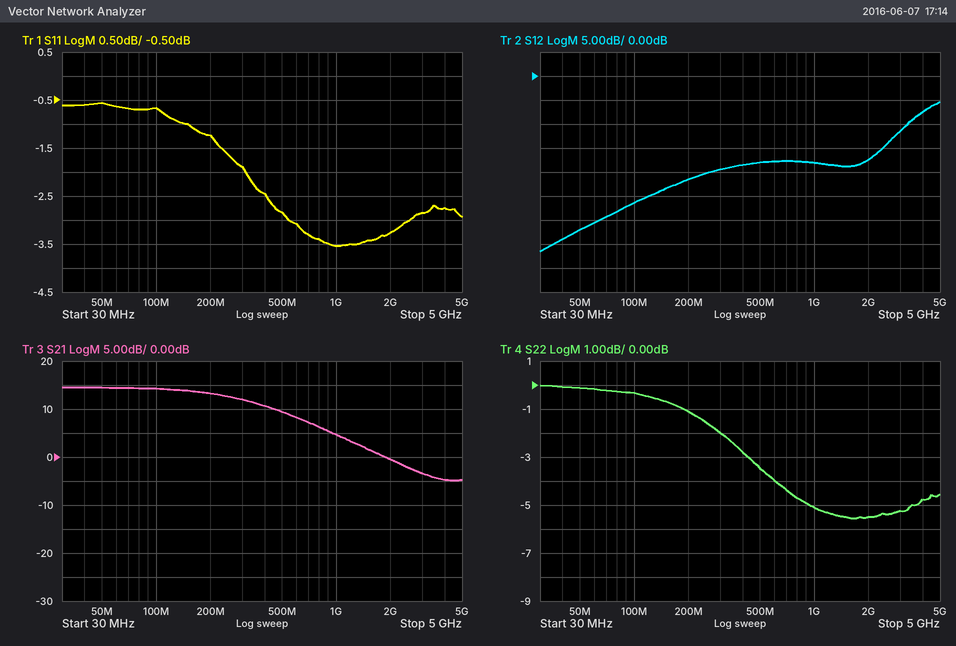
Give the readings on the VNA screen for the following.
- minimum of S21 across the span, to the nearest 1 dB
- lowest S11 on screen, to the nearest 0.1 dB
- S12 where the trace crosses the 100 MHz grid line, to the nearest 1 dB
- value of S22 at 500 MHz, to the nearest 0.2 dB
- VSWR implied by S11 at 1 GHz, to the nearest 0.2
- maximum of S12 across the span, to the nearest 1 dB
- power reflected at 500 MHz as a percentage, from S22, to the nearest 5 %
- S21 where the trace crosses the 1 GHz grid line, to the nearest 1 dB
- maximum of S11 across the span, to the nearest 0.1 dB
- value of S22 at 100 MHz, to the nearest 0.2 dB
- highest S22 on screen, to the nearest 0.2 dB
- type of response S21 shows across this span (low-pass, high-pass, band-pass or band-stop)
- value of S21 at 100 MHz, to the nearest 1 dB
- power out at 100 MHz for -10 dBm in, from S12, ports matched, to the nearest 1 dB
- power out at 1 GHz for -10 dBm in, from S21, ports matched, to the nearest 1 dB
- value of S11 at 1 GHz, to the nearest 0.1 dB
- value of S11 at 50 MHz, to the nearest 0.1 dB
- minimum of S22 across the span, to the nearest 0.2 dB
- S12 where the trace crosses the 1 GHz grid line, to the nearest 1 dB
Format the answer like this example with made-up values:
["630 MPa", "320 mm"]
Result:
["-5 dB", "-3.5 dB", "-26 dB", "-3.4 dB", "5.0", "-5 dB", "45 %", "5 dB", "-0.6 dB", "-0.4 dB", "0.0 dB", "low-pass", "14 dB", "-36 dBm", "-5 dBm", "-3.5 dB", "-0.6 dB", "-5.6 dB", "-18 dB"]
